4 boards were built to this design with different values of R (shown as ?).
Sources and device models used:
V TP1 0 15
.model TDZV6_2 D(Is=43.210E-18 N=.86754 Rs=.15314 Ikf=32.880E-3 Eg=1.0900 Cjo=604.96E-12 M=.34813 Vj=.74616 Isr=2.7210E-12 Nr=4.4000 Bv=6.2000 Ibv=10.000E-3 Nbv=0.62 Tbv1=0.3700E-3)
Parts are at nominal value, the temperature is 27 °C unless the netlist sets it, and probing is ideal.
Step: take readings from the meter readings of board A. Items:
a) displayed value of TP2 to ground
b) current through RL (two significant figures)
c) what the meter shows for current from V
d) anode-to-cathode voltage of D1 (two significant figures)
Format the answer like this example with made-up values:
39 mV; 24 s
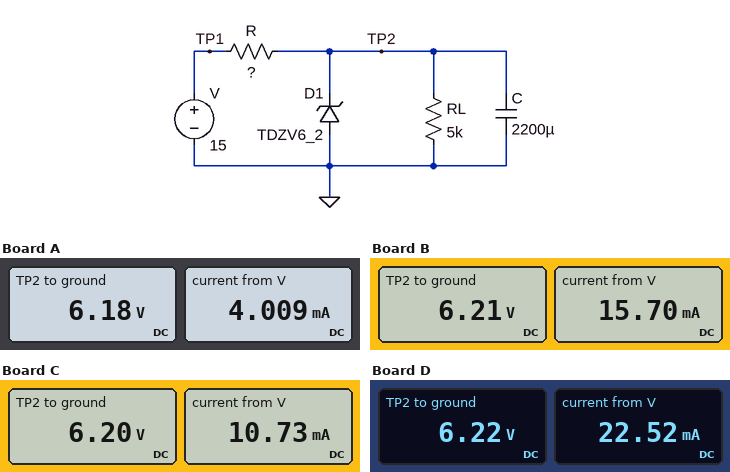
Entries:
6.18 V; 1.2 mA; 4.009 mA; -6.2 V
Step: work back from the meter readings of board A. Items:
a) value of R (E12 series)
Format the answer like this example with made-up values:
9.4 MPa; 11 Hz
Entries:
2.2 kΩ
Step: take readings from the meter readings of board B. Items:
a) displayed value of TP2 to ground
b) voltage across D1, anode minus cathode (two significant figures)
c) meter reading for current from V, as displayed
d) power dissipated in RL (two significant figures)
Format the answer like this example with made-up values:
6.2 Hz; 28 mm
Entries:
6.21 V; -6.2 V; 15.70 mA; 7.7 mW
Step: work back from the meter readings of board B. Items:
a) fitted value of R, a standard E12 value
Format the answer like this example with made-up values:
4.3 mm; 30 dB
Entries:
560 Ω
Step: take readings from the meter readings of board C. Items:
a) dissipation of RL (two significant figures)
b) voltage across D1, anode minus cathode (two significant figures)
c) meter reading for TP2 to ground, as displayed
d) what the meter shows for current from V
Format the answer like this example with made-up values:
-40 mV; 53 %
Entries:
7.7 mW; -6.2 V; 6.20 V; 10.73 mA
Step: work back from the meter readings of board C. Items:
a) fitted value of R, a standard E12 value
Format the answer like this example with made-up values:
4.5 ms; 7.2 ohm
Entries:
820 Ω
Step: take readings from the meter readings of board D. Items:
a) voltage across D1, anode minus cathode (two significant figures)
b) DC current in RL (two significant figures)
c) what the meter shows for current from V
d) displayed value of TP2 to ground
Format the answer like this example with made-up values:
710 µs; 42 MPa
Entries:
-6.2 V; 1.2 mA; 22.52 mA; 6.22 V
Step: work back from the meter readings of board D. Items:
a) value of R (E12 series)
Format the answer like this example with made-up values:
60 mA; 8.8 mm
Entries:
390 Ω
